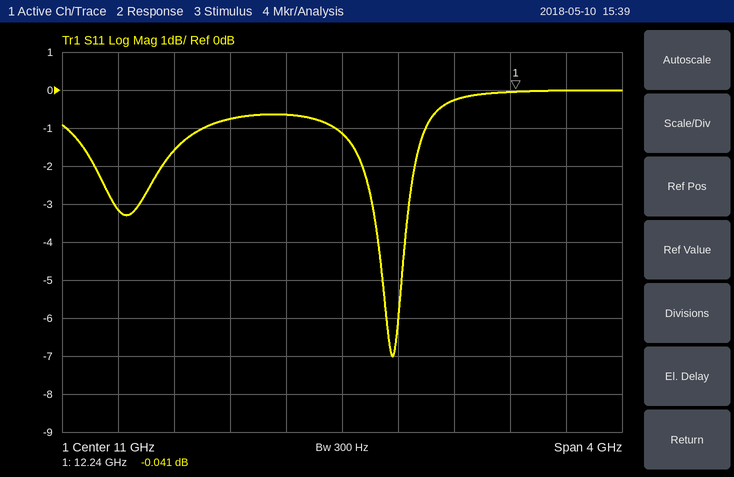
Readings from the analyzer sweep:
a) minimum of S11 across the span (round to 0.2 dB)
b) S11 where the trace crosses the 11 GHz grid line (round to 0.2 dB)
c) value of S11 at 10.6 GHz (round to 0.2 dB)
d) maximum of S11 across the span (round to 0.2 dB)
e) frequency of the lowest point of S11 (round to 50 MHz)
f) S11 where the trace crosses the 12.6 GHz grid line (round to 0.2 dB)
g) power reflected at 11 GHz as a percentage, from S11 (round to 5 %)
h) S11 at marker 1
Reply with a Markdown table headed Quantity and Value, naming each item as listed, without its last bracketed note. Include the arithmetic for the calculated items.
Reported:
| Quantity | Value |
|---|---|
| minimum of S11 across the span | -7.0 dB |
| S11 where the trace crosses the 11 GHz grid line | -1.2 dB |
| value of S11 at 10.6 GHz | -0.6 dB |
| maximum of S11 across the span | 0.0 dB |
| frequency of the lowest point of S11 | 11.35 GHz |
| S11 where the trace crosses the 12.6 GHz grid line | 0.0 dB |
| power reflected at 11 GHz as a percentage, from S11 | 10^(-1.2/10) ≈ 75.9 %, so 75 % to the nearest 5 % |
| S11 at marker 1 | -0.041 dB |
